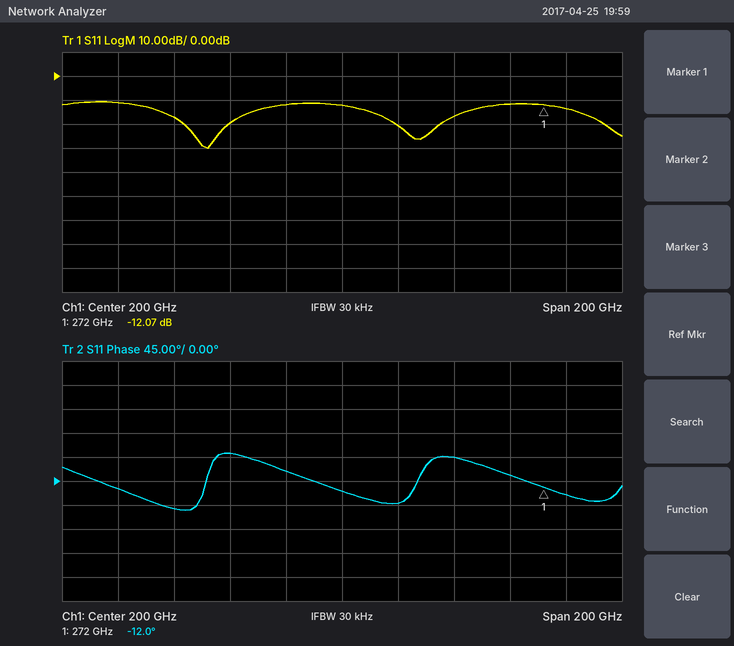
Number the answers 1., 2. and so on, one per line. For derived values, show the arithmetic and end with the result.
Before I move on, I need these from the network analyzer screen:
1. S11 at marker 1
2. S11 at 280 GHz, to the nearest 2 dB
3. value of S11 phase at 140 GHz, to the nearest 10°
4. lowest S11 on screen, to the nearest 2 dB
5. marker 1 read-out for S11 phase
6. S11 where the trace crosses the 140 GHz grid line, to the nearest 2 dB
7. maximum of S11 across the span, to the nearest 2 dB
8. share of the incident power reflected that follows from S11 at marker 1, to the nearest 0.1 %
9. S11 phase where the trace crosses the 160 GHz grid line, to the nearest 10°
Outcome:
1. -12.07 dB
2. -14 dB
3. -50°
4. -30 dB
5. -12.0°
6. -18 dB
7. -10 dB
8. 10^(-12.07/10) ≈ 6.2 %
9. 50°
